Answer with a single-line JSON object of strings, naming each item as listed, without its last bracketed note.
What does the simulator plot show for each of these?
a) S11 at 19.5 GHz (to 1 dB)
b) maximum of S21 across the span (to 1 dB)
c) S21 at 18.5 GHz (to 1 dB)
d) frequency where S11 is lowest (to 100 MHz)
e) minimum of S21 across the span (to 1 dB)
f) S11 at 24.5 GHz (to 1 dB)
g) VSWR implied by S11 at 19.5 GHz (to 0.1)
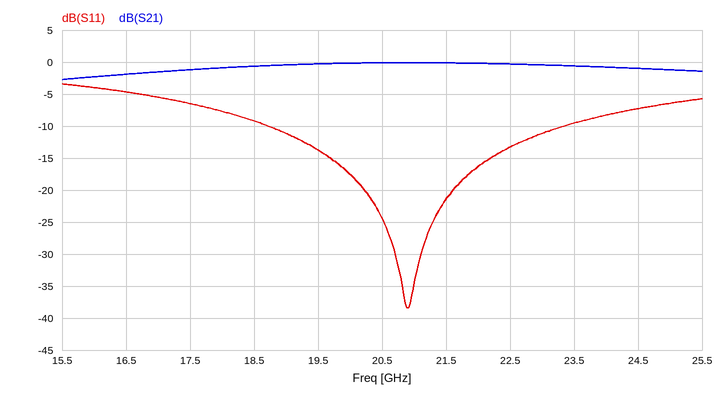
{"S11 at 19.5 GHz": "-14 dB", "maximum of S21 across the span": "0 dB", "S21 at 18.5 GHz": "-1 dB", "frequency where S11 is lowest": "20.9 GHz", "minimum of S21 across the span": "-3 dB", "S11 at 24.5 GHz": "-7 dB", "VSWR implied by S11 at 19.5 GHz": "1.5"}
